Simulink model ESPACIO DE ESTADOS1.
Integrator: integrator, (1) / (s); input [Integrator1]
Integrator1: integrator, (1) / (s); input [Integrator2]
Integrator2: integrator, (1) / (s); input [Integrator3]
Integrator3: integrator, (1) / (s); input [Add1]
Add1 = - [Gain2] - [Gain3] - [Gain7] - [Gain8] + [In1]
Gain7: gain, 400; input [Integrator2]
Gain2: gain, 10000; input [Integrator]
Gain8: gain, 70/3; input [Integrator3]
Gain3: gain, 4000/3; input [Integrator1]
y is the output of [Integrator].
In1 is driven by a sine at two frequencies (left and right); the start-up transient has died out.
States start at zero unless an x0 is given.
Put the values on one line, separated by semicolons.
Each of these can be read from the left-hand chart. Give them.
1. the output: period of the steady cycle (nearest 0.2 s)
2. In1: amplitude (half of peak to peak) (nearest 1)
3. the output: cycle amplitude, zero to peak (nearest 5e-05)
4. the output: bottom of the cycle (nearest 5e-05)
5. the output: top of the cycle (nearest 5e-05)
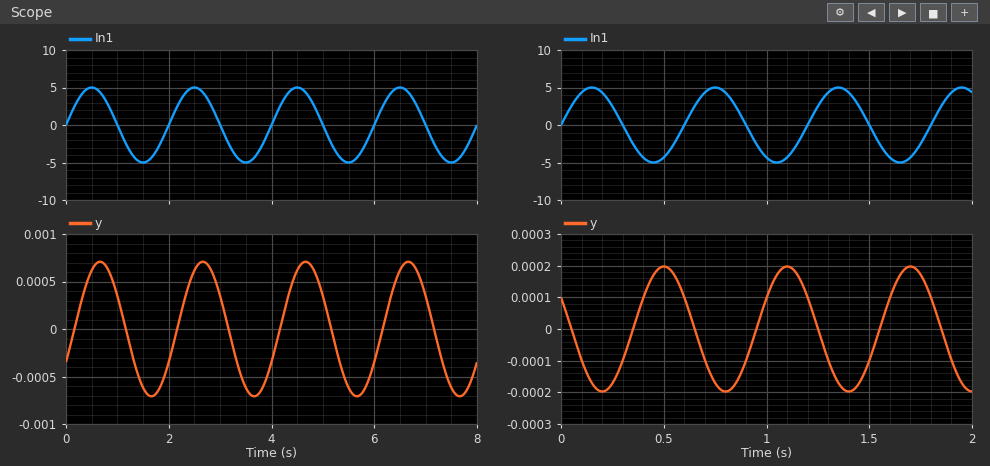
2.0 s; 5; 0.00070; -0.00070; 0.00070
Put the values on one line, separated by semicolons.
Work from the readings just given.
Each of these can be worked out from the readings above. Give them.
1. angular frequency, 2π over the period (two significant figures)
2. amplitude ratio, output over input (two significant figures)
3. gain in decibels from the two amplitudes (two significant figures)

3.1 rad/s; 0.00014; -77 dB
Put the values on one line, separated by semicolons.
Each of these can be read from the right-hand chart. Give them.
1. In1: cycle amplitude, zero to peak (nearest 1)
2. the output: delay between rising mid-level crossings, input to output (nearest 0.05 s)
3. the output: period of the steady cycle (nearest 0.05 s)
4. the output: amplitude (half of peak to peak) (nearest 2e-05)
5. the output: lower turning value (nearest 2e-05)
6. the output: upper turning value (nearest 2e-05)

5; 0.35 s; 0.60 s; 0.00020; -0.00020; 0.00020
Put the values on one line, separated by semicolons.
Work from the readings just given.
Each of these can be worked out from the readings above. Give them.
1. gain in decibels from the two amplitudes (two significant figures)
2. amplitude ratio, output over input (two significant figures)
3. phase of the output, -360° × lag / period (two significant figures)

-88 dB; 0.000040; -210°
